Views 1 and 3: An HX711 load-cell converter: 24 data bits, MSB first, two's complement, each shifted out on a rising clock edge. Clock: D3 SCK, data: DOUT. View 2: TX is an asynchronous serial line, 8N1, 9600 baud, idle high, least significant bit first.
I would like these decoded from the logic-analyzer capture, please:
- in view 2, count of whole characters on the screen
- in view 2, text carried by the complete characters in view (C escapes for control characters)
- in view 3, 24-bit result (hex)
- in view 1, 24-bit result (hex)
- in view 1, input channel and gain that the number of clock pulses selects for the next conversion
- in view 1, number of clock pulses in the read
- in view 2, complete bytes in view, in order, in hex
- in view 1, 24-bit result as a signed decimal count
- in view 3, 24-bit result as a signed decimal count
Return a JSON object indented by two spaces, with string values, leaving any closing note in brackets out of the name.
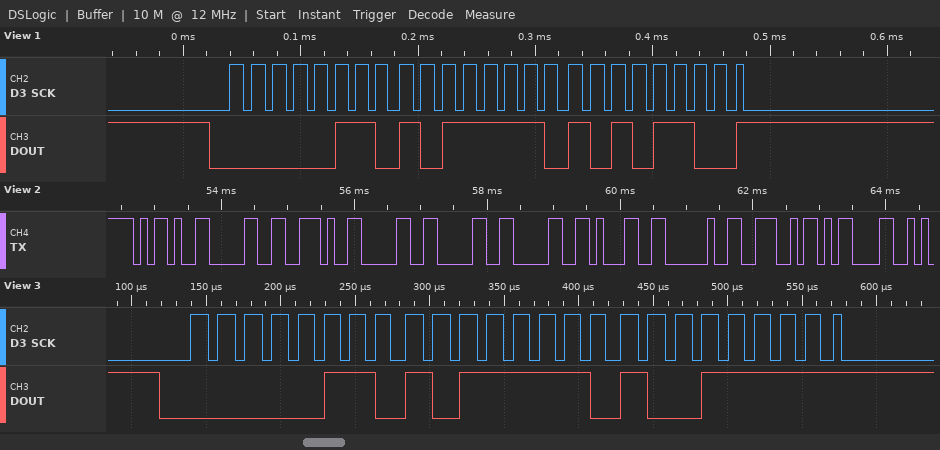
{
  "in view 2, count of whole characters on the screen": "10",
  "in view 2, text carried by the complete characters in view": "\"-0.0001 N\\r\"",
  "in view 3, 24-bit result": "0x06BE9F",
  "in view 1, 24-bit result": "0x06BEAC",
  "in view 1, input channel and gain that the number of clock pulses selects for the next conversion": "channel A, gain 128",
  "in view 1, number of clock pulses in the read": "25",
  "in view 2, complete bytes in view, in order, in hex": "0x2D 0x30 0x2E 0x30 0x30 0x30 0x31 0x20 0x4E 0x0D",
  "in view 1, 24-bit result as a signed decimal count": "442028",
  "in view 3, 24-bit result as a signed decimal count": "442015"
}
